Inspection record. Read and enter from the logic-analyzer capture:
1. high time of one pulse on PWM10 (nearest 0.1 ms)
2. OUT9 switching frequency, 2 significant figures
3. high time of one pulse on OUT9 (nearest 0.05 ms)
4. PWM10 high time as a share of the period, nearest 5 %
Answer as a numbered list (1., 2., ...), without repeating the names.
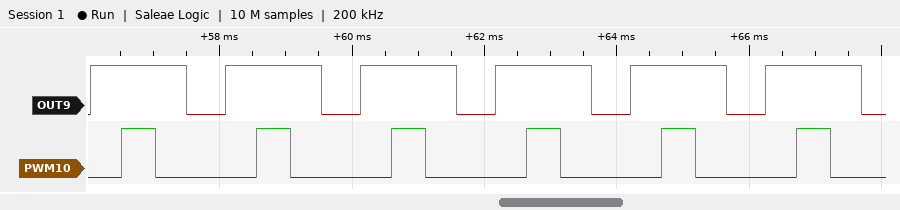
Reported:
1. 0.5 ms
2. 490 Hz
3. 1.45 ms
4. 25 %
